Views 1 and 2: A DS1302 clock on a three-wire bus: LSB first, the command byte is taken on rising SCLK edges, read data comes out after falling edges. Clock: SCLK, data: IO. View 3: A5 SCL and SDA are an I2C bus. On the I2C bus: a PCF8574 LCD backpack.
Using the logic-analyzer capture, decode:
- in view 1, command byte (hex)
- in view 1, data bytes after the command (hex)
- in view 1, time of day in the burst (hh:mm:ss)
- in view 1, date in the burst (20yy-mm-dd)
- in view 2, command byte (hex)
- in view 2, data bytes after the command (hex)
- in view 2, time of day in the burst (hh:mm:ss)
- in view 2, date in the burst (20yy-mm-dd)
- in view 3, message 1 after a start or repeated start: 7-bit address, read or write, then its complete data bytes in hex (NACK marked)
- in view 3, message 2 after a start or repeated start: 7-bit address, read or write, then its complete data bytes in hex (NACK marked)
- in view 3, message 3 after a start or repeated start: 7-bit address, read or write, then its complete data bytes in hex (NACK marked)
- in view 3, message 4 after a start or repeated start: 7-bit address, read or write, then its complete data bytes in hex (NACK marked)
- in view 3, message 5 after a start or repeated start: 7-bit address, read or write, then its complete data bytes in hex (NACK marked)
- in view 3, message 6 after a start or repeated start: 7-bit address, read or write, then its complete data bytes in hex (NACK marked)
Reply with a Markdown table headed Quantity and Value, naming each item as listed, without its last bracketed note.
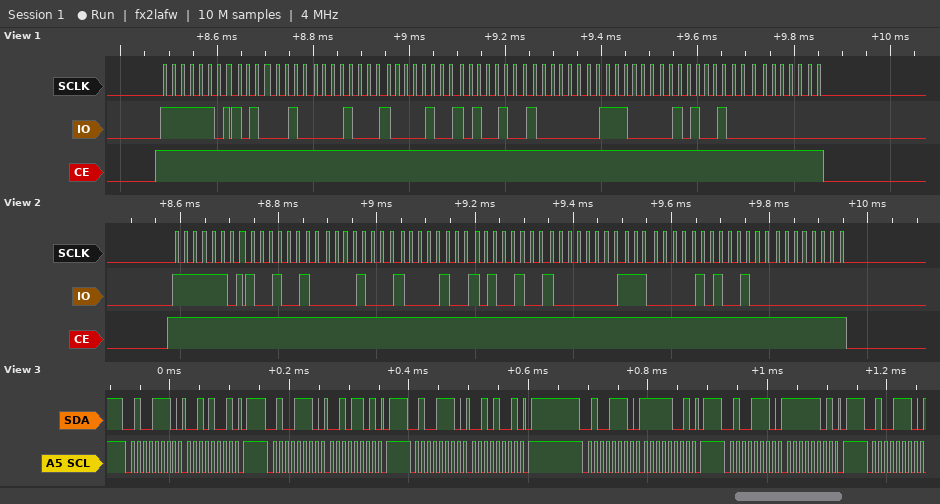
| Quantity | Value |
|---|---|
| in view 1, command byte | 0xBF |
| in view 1, data bytes after the command | 45 10 21 25 01 07 25 00 |
| in view 1, time of day in the burst | 21:10:45 |
| in view 1, date in the burst | 2025-01-25 |
| in view 2, command byte | 0xBF |
| in view 2, data bytes after the command | 49 10 21 25 01 07 25 00 |
| in view 2, time of day in the burst | 21:10:49 |
| in view 2, date in the burst | 2025-01-25 |
| in view 3, message 1 after a start or repeated start: 7-bit address, read or write, then its complete data bytes in hex | 0x27 write: 29 |
| in view 3, message 2 after a start or repeated start: 7-bit address, read or write, then its complete data bytes in hex | 0x27 write: 2D |
| in view 3, message 3 after a start or repeated start: 7-bit address, read or write, then its complete data bytes in hex | 0x27 write: 29 |
| in view 3, message 4 after a start or repeated start: 7-bit address, read or write, then its complete data bytes in hex | 0x27 write: F9 |
| in view 3, message 5 after a start or repeated start: 7-bit address, read or write, then its complete data bytes in hex | 0x27 write: FD |
| in view 3, message 6 after a start or repeated start: 7-bit address, read or write, then its complete data bytes in hex | 0x27 write |
